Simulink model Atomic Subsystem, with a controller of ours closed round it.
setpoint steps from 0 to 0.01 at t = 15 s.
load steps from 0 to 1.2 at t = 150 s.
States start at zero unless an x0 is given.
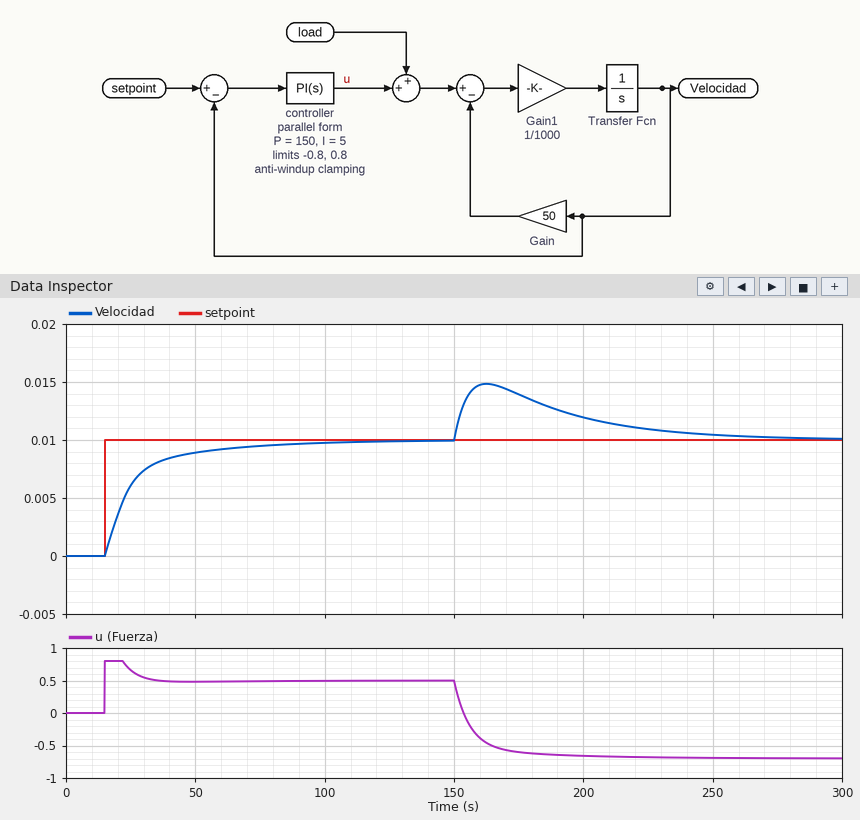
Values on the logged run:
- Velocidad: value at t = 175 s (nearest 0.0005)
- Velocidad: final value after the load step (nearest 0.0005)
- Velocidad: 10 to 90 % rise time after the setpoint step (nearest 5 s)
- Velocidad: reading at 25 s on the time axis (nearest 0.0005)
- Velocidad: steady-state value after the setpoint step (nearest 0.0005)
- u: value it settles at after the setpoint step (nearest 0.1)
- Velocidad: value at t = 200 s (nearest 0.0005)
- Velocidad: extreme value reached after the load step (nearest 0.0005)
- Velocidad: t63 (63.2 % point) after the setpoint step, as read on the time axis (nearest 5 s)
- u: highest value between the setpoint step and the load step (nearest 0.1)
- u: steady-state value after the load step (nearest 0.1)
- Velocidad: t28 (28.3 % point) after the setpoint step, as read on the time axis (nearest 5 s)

0.0140
0.0100
35 s
0.0060
0.0100
0.5
0.0120
0.0150
25 s
0.8
-0.7
20 s
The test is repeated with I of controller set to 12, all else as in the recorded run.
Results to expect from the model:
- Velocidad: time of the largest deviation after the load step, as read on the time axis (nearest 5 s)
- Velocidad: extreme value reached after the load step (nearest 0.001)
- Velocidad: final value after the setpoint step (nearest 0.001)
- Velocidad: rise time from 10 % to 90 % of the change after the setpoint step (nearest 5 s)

160 s
0.014
0.010
20 s
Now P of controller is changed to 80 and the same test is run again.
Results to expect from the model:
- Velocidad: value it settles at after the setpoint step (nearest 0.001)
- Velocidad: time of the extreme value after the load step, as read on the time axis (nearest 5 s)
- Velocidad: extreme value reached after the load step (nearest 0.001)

0.010
165 s
0.017
